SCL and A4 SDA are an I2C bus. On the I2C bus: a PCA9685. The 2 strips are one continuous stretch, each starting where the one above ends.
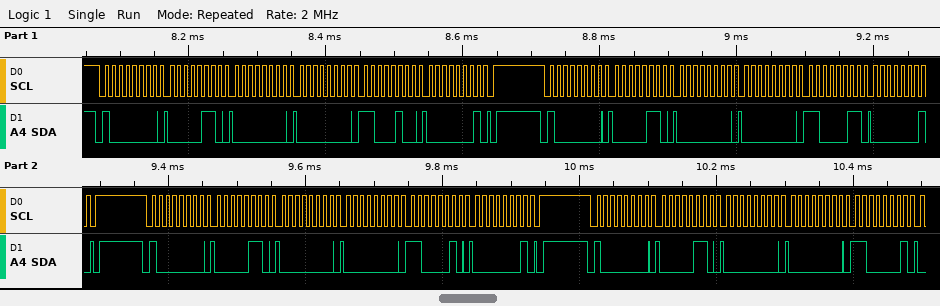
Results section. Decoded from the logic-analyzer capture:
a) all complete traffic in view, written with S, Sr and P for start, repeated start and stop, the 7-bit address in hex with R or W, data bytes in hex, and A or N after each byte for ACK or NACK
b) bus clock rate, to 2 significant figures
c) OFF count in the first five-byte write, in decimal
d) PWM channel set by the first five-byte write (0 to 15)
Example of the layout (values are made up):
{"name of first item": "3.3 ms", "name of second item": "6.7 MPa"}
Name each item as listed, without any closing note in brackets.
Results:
{"all complete traffic in view, written with S, Sr and P for start, repeated start and stop, the 7-bit address in hex with R or W, data bytes in hex, and A or N after each byte for ACK or NACK": "S 40W A 06 A 00 A 00 A C4 A 01 A P S 40W A 06 A 00 A 00 A C3 A 01 A P S 40W A 06 A 00 A 00 A C2 A 01 A P S 40W A 06 A 00 A 00 A C1 A", "bus clock rate, to 2 significant figures": "100 kHz", "OFF count in the first five-byte write, in decimal": "452", "PWM channel set by the first five-byte write": "0"}
